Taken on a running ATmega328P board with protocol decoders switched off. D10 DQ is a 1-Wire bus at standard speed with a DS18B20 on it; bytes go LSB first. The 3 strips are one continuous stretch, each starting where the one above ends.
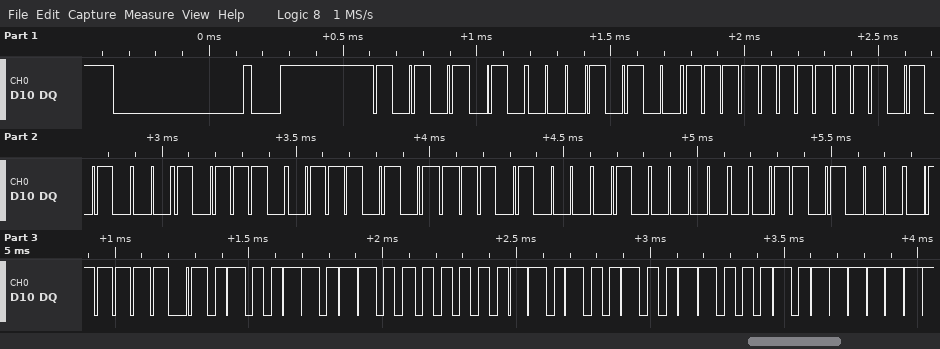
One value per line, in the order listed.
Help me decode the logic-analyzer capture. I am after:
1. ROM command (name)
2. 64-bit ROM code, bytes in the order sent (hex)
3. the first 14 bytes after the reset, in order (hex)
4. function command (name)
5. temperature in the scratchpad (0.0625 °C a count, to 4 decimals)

Match ROM
28 FF 57 74 AE 17 02 16
55 28 FF 57 74 AE 17 02 16 BE B2 01 4B 46
Read Scratchpad
27.1250 °C
